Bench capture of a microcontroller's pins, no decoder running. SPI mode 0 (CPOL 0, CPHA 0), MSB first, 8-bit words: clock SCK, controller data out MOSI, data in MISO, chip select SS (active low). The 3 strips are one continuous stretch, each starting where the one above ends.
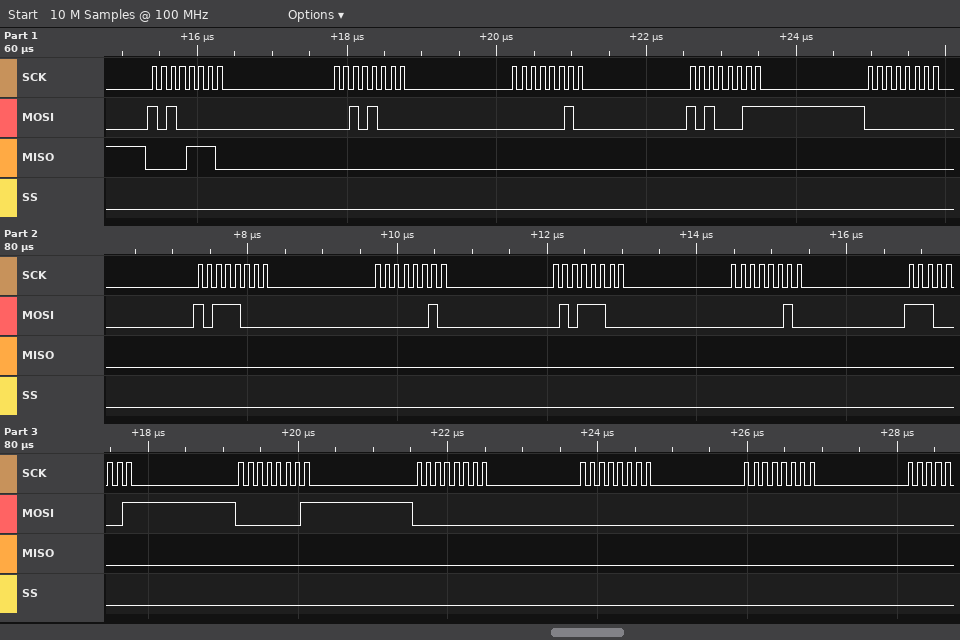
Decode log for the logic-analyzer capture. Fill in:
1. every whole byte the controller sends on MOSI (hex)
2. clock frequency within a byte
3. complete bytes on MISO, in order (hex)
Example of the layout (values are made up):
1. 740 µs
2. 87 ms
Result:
1. A0 28 02 A3 00 B8 02 5C 02 E1 01 00 00 00
2. 8 MHz
3. 0E 00 00 00 00 00 00 00 00 00 00 00 00 00
